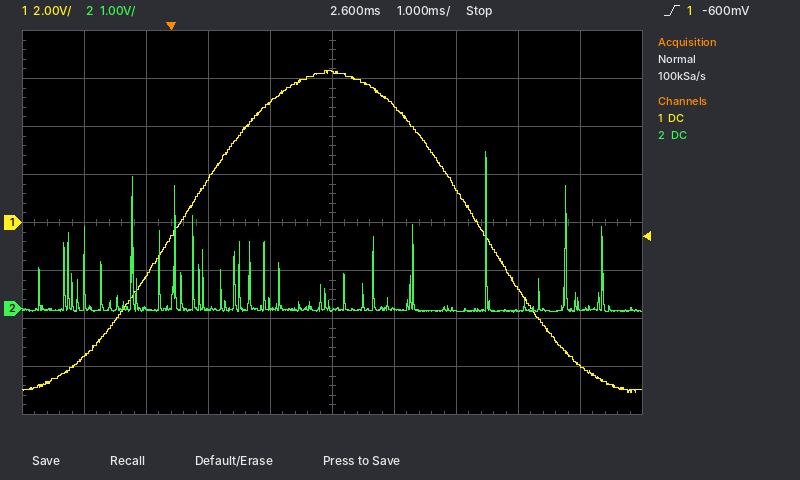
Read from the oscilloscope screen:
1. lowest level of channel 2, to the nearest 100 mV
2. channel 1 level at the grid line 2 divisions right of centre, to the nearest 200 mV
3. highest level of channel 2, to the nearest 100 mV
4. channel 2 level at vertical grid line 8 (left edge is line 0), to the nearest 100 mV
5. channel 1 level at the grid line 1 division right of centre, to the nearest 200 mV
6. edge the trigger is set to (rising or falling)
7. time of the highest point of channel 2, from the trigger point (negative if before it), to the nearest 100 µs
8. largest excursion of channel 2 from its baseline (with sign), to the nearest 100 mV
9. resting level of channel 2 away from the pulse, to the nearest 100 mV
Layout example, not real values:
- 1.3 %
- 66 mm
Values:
- -100 mV
- 1.4 V
- 3.3 V
- 0.0 V
- 4.8 V
- rising
- +5.1 ms
- +3.3 V
- 0.0 V
